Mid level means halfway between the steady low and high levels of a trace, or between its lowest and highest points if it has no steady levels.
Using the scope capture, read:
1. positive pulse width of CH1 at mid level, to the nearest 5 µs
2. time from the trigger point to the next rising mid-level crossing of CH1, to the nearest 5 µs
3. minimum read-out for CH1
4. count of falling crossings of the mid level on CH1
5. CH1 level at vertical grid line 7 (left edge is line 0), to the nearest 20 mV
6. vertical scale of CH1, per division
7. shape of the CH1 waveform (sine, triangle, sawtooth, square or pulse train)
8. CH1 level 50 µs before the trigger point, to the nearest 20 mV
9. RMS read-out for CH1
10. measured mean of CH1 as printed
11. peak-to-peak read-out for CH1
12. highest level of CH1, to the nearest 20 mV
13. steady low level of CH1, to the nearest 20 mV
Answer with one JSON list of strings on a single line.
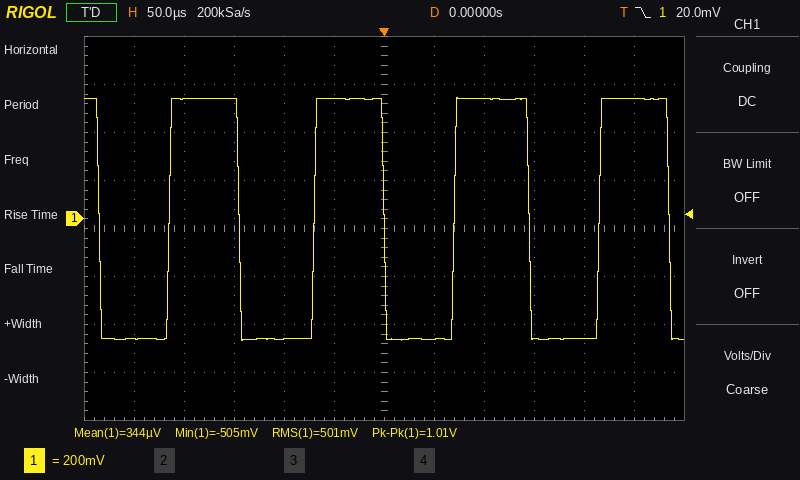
["70 µs", "70 µs", "-505 mV", "5", "-500 mV", "200 mV", "square", "500 mV", "501 mV", "344 µV", "1.01 V", "500 mV", "-500 mV"]
